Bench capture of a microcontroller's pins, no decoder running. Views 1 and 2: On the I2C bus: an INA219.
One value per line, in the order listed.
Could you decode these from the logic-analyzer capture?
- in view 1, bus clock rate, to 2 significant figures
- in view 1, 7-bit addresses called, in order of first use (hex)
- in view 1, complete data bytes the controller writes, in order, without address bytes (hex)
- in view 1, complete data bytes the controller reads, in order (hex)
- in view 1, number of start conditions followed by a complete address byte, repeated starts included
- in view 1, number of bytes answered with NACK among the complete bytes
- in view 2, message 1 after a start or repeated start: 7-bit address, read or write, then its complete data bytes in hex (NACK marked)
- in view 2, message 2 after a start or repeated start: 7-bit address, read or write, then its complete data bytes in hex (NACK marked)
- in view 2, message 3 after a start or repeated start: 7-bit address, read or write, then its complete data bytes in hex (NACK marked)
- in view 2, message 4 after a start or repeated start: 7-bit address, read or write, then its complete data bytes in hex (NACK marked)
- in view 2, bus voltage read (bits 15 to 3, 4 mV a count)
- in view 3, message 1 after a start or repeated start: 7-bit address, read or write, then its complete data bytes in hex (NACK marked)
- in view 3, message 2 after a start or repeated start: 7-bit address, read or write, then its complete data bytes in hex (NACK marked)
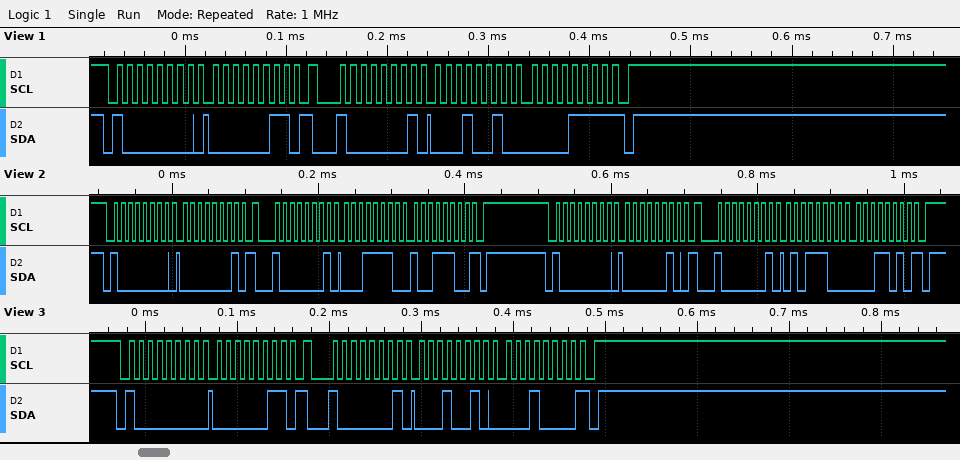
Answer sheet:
100 kHz
0x40
03
12 0F
2
1
0x40 write: 01
0x40 read: 1E 9C NACK
0x40 write: 02
0x40 read: 5C 1A NACK
11.788 V
0x40 write: 03
0x40 read: 12 10 NACK
